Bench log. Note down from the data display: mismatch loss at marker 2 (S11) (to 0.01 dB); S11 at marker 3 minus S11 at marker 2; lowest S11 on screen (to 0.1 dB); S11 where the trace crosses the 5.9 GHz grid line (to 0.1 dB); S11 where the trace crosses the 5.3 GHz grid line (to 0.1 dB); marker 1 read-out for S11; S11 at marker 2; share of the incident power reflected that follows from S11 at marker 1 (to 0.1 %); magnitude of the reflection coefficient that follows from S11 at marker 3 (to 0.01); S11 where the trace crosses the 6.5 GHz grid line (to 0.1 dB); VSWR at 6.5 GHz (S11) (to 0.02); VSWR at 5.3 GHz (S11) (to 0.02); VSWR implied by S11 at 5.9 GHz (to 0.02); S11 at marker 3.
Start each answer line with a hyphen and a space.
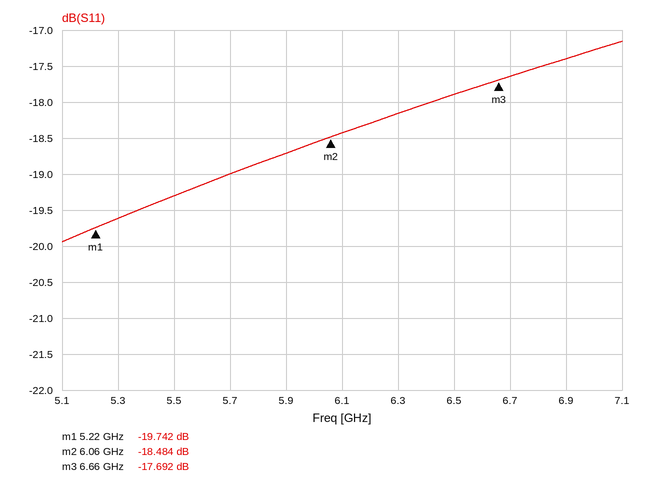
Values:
- 0.06 dB
- 0.792 dB
- -19.9 dB
- -18.7 dB
- -19.6 dB
- -19.742 dB
- -18.484 dB
- 1.1 %
- 0.13
- -17.9 dB
- 1.30
- 1.24
- 1.26
- -17.692 dB
